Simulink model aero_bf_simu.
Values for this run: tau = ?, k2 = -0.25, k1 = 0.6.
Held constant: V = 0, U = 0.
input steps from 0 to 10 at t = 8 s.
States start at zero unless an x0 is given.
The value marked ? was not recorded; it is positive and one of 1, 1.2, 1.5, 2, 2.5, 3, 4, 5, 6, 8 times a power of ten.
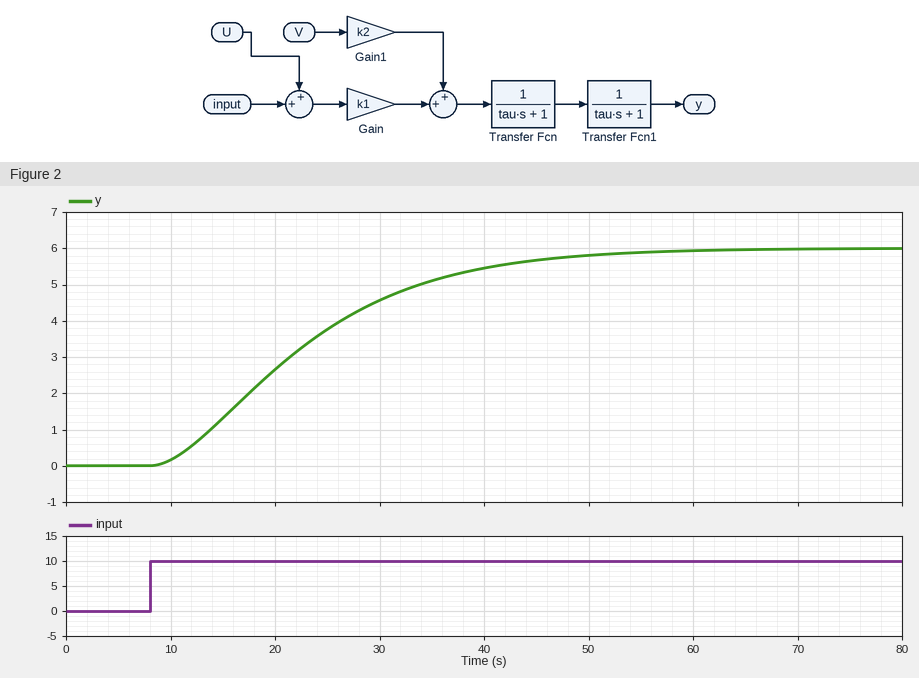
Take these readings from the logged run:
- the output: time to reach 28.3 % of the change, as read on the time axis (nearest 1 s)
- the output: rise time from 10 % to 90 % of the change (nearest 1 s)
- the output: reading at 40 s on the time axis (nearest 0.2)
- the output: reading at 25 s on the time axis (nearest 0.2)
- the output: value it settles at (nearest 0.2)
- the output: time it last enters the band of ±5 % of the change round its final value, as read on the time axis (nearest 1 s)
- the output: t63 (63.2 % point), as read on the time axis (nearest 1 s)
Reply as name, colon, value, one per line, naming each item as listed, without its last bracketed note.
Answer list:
the output: time to reach 28.3 % of the change, as read on the time axis: 16 s
the output: rise time from 10 % to 90 % of the change: 27 s
the output: reading at 40 s on the time axis: 5.4
the output: reading at 25 s on the time axis: 3.8
the output: value it settles at: 6.0
the output: time it last enters the band of ±5 % of the change round its final value, as read on the time axis: 46 s
the output: t63 (63.2 % point), as read on the time axis: 25 s
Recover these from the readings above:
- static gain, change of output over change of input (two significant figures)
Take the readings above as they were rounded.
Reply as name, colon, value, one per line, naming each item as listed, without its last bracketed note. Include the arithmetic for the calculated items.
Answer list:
static gain, change of output over change of input: (6 - 0) / (10 - 0) = 0.60
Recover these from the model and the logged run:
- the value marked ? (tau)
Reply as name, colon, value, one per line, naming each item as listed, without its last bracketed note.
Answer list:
the value marked ?: 8
